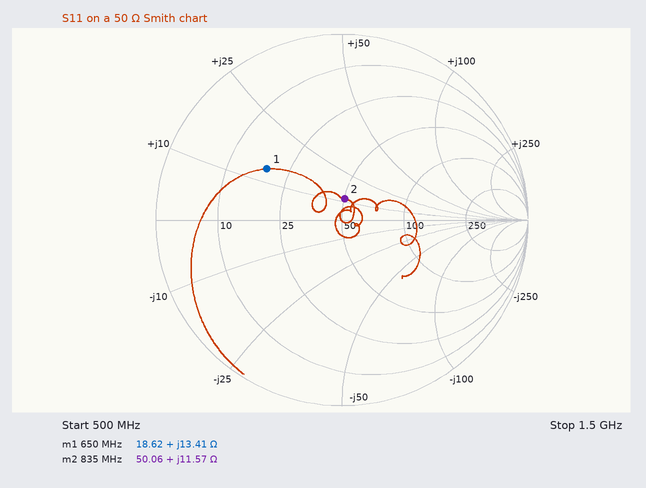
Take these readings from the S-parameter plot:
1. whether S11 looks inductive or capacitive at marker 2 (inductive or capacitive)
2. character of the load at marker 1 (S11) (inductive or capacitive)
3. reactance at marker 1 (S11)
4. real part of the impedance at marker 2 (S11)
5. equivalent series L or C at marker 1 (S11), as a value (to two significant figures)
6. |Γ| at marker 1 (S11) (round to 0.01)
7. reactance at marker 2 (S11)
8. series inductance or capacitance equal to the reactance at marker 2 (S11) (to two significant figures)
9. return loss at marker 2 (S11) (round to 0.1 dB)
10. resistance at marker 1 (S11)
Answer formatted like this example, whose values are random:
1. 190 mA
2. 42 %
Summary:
1. inductive
2. inductive
3. +13.41 Ω
4. 50.06 Ω
5. 3.3 nH
6. 0.49
7. +11.57 Ω
8. 2.2 nH
9. 18.8 dB
10. 18.62 Ω
